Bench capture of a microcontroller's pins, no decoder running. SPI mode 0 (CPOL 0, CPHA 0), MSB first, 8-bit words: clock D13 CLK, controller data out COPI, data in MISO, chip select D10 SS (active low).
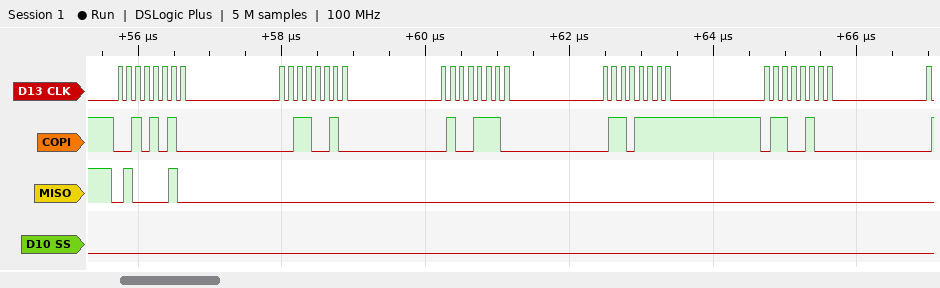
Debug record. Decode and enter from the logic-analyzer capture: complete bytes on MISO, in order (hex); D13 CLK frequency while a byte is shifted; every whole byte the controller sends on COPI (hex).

42 00 00 00 00
8 MHz
2A 32 4E 6F 64
